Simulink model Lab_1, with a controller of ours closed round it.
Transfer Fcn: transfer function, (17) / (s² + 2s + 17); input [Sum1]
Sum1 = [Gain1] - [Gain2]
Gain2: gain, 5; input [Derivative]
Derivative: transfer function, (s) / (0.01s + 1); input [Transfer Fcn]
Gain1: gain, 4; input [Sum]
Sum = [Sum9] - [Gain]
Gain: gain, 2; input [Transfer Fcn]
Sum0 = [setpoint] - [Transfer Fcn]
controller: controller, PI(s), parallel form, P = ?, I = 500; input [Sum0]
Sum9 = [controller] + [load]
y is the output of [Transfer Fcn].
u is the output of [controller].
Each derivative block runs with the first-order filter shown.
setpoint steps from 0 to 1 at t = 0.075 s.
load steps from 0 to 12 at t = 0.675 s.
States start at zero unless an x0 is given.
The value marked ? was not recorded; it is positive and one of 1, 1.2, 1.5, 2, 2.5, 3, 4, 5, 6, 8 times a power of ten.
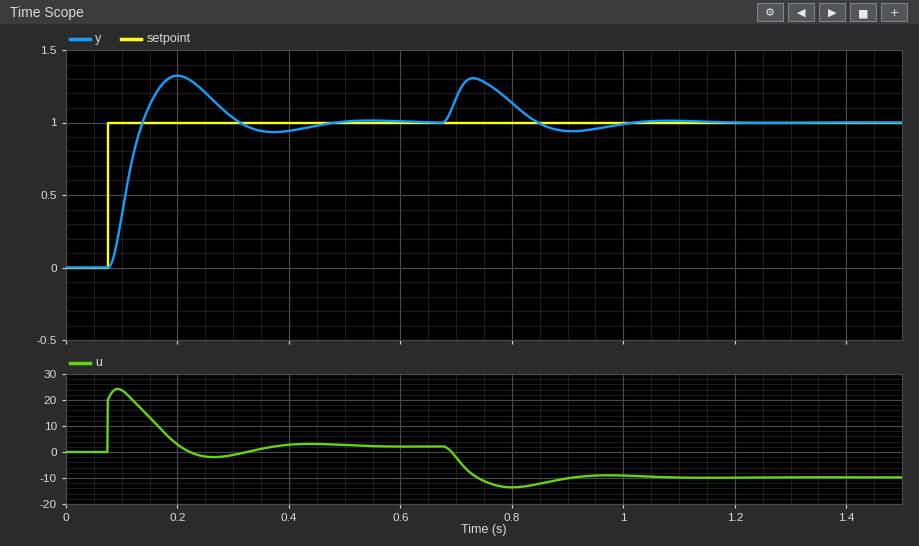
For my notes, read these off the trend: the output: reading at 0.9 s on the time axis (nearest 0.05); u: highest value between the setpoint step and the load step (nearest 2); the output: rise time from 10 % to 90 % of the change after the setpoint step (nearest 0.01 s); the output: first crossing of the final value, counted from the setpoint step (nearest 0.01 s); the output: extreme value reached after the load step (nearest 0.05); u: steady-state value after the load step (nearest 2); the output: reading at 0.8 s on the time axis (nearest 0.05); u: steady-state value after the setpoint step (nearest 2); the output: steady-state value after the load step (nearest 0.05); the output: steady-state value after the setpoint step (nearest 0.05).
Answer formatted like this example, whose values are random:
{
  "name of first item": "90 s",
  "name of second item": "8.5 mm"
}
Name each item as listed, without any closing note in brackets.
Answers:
{
  "the output: reading at 0.9 s on the time axis": "0.95",
  "u: highest value between the setpoint step and the load step": "24",
  "the output: rise time from 10 % to 90 % of the change after the setpoint step": "0.04 s",
  "the output: first crossing of the final value, counted from the setpoint step": "0.06 s",
  "the output: extreme value reached after the load step": "1.30",
  "u: steady-state value after the load step": "-10",
  "the output: reading at 0.8 s on the time axis": "1.15",
  "u: steady-state value after the setpoint step": "2",
  "the output: steady-state value after the load step": "1.00",
  "the output: steady-state value after the setpoint step": "1.00"
}
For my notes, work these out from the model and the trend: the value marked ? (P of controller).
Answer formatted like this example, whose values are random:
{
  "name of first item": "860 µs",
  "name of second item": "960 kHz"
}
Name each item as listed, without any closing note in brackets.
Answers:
{
  "the value marked ?": "20"
}
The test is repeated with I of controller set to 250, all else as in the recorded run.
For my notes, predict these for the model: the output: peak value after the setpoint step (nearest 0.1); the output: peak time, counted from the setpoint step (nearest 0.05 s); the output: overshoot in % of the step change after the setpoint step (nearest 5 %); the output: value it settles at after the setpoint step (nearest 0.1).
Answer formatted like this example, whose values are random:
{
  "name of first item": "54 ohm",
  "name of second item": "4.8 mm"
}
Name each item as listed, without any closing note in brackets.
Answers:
{
  "the output: peak value after the setpoint step": "1.2",
  "the output: peak time, counted from the setpoint step": "0.15 s",
  "the output: overshoot in % of the step change after the setpoint step": "20 %",
  "the output: value it settles at after the setpoint step": "1.0"
}
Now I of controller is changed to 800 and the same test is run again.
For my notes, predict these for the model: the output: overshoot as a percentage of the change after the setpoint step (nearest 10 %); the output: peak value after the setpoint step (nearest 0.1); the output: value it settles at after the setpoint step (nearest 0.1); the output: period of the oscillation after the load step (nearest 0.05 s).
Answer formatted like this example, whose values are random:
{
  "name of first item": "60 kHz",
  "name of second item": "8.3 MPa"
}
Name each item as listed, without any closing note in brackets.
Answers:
{
  "the output: overshoot as a percentage of the change after the setpoint step": "40 %",
  "the output: peak value after the setpoint step": "1.4",
  "the output: value it settles at after the setpoint step": "1.0",
  "the output: period of the oscillation after the load step": "0.25 s"
}
